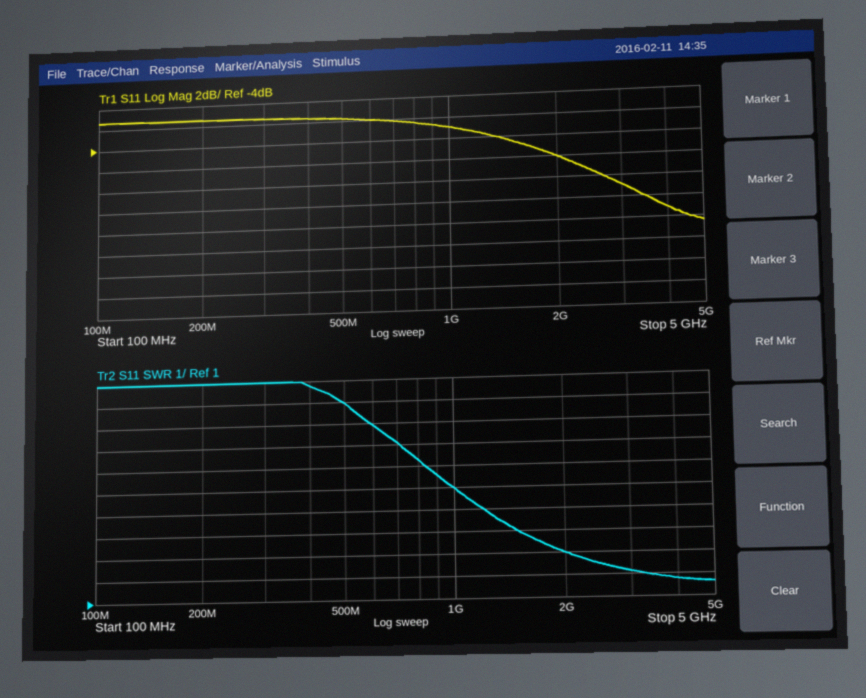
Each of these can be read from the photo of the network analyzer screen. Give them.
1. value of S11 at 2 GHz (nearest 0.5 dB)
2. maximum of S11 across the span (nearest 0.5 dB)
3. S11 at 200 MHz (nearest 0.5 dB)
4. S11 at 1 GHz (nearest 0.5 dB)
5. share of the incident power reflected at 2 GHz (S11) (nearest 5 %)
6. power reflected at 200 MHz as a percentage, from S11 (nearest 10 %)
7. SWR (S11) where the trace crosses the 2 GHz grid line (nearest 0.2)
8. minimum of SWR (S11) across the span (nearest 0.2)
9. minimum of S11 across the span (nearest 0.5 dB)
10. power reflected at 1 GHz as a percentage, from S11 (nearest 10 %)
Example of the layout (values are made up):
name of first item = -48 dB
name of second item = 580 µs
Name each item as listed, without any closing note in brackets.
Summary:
value of S11 at 2 GHz = -6.0 dB
maximum of S11 across the span = -1.5 dB
S11 at 200 MHz = -1.5 dB
S11 at 1 GHz = -3.0 dB
share of the incident power reflected at 2 GHz (S11) = 25 %
power reflected at 200 MHz as a percentage, from S11 = 70 %
SWR (S11) where the trace crosses the 2 GHz grid line = 3.0
minimum of SWR (S11) across the span = 1.6
minimum of S11 across the span = -12.5 dB
power reflected at 1 GHz as a percentage, from S11 = 50 %
